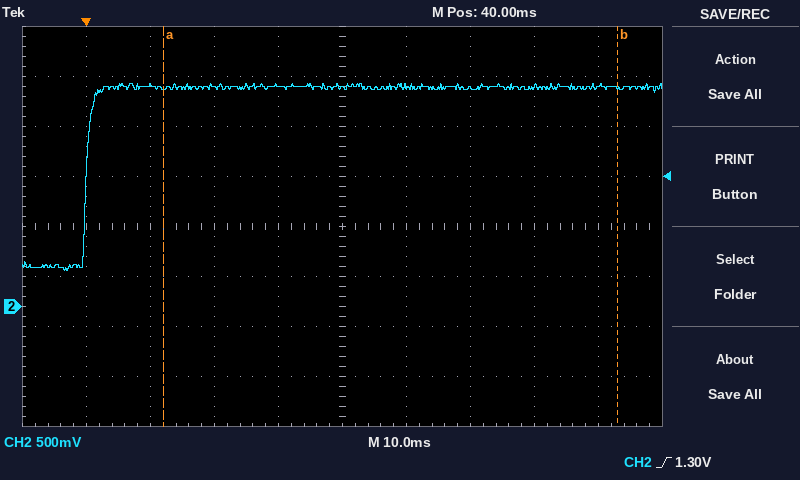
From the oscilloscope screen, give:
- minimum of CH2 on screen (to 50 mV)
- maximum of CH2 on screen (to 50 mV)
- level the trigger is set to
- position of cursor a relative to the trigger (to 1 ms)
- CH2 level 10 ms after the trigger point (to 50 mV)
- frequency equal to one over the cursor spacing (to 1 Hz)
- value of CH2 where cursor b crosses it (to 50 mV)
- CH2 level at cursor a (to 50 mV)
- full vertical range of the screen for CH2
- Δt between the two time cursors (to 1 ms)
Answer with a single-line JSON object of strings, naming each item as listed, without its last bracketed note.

{"minimum of CH2 on screen": "350 mV", "maximum of CH2 on screen": "2.25 V", "level the trigger is set to": "1.30 V", "position of cursor a relative to the trigger": "+12 ms", "CH2 level 10 ms after the trigger point": "2.20 V", "frequency equal to one over the cursor spacing": "14 Hz", "value of CH2 where cursor b crosses it": "2.20 V", "CH2 level at cursor a": "2.20 V", "full vertical range of the screen for CH2": "4 V", "Δt between the two time cursors": "71 ms"}
